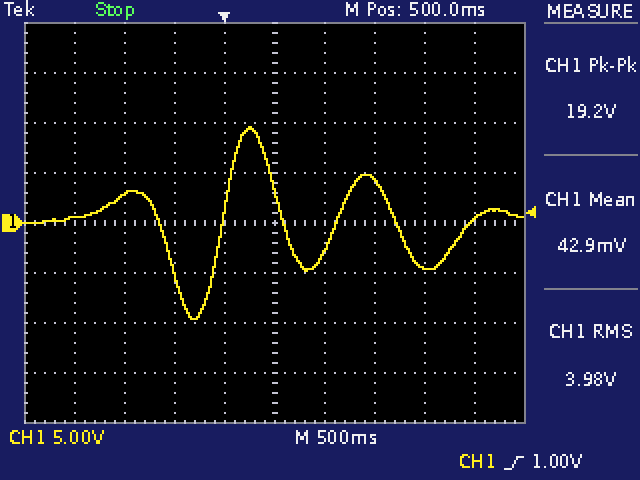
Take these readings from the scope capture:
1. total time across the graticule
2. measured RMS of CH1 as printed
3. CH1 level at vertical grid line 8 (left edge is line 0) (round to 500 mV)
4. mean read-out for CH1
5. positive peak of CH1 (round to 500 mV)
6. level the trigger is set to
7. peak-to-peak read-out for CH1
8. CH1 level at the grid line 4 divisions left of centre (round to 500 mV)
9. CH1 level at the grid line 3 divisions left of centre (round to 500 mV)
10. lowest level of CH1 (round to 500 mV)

5 s
3.98 V
-4.5 V
42.9 mV
9.5 V
1.00 V
19.2 V
500 mV
3.0 V
-9.5 V
